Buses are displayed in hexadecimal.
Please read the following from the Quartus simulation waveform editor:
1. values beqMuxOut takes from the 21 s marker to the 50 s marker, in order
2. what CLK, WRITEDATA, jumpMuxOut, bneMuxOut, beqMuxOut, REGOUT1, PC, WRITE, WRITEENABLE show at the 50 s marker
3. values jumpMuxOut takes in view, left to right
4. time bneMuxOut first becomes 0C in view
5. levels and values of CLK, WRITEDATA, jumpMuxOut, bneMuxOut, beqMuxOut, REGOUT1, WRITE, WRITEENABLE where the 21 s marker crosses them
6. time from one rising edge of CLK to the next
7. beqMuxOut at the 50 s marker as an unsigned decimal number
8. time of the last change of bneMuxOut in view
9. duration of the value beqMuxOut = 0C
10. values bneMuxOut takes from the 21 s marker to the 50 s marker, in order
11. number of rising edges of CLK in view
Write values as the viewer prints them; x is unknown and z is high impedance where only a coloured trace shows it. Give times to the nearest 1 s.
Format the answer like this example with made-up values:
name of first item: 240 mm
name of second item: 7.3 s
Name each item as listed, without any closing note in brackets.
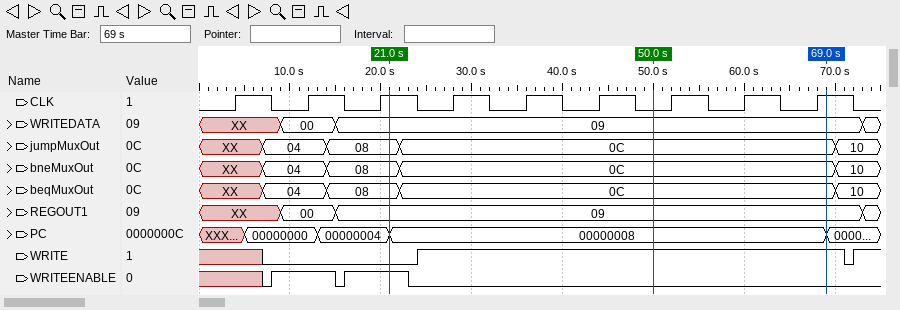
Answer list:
values beqMuxOut takes from the 21 s marker to the 50 s marker, in order: 08, 0C
what CLK, WRITEDATA, jumpMuxOut, bneMuxOut, beqMuxOut, REGOUT1, PC, WRITE, WRITEENABLE show at the 50 s marker: CLK=0, WRITEDATA=09, jumpMuxOut=0C, bneMuxOut=0C, beqMuxOut=0C, REGOUT1=09, PC=00000008, WRITE=1, WRITEENABLE=0
values jumpMuxOut takes in view, left to right: XX, 04, 08, 0C, 10
time bneMuxOut first becomes 0C in view: 22 s
levels and values of CLK, WRITEDATA, jumpMuxOut, bneMuxOut, beqMuxOut, REGOUT1, WRITE, WRITEENABLE where the 21 s marker crosses them: CLK=1, WRITEDATA=09, jumpMuxOut=08, bneMuxOut=08, beqMuxOut=08, REGOUT1=09, WRITE=0, WRITEENABLE=1
time from one rising edge of CLK to the next: 8 s
beqMuxOut at the 50 s marker as an unsigned decimal number: 12
time of the last change of bneMuxOut in view: 70 s
duration of the value beqMuxOut = 0C: 48 s
values bneMuxOut takes from the 21 s marker to the 50 s marker, in order: 08, 0C
number of rising edges of CLK in view: 9
